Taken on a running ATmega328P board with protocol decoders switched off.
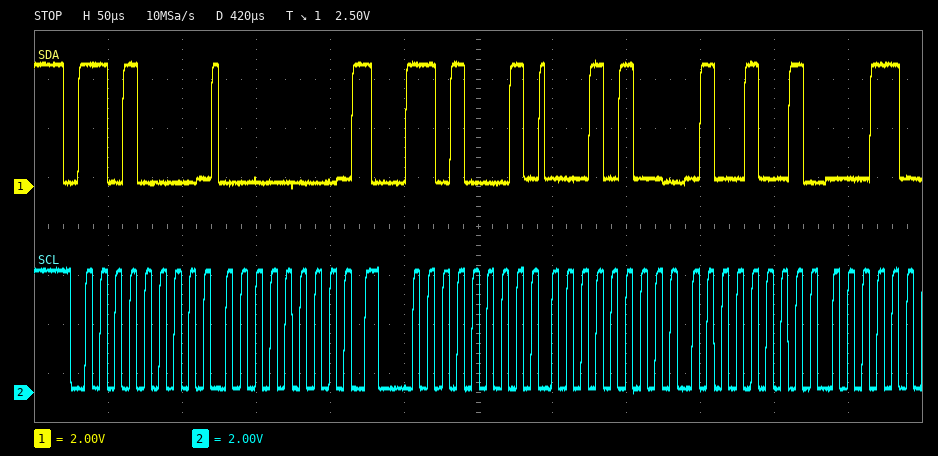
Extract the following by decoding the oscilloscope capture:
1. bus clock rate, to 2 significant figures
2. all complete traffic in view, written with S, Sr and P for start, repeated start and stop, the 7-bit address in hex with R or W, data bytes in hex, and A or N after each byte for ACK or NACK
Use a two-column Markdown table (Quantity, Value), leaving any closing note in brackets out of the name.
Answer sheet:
| Quantity | Value |
|---|---|
| bus clock rate, to 2 significant figures | 100 kHz |
| all complete traffic in view, written with S, Sr and P for start, repeated start and stop, the 7-bit address in hex with R or W, data bytes in hex, and A or N after each byte for ACK or NACK | S 68W A 00 A Sr 68R A 14 A 49 A |
